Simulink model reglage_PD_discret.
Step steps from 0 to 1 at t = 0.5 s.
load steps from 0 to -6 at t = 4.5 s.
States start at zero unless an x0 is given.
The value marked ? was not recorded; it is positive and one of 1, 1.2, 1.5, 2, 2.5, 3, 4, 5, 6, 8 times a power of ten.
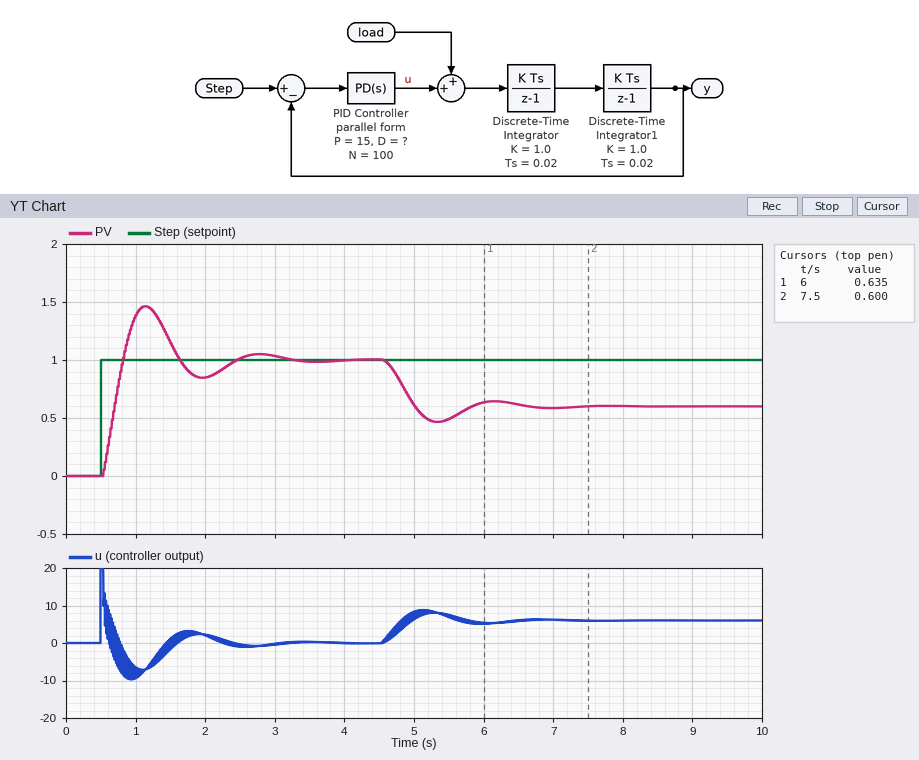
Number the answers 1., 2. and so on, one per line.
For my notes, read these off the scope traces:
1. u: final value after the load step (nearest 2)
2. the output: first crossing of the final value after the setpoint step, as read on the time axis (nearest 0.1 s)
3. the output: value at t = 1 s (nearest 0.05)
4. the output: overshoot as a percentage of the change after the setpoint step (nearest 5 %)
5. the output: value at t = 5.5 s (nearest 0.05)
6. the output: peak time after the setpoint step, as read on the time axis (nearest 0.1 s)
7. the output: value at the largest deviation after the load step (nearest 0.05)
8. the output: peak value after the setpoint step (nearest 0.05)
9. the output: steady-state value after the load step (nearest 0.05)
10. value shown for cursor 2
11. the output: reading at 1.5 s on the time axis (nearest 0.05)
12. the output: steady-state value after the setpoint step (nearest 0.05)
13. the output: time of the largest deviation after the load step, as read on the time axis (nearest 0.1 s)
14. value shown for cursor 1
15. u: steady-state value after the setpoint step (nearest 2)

1. 6
2. 0.8 s
3. 1.40
4. 45 %
5. 0.50
6. 1.1 s
7. 0.45
8. 1.45
9. 0.60
10. 0.600
11. 1.15
12. 1.00
13. 5.3 s
14. 0.635
15. 0
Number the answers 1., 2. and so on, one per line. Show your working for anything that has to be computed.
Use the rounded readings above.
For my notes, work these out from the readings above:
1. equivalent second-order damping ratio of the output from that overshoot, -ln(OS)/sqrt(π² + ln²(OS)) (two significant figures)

1. ln(0.45) = -0.799; 0.799 / sqrt(9.870 + 0.638) = 0.25
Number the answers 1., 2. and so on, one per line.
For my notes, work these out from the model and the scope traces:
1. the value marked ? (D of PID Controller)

1. 1.2
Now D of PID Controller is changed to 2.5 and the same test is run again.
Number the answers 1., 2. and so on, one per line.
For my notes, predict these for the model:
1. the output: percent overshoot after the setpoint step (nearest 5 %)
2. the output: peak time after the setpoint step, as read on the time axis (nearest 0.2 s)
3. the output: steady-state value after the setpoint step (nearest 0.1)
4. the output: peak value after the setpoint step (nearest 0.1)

1. 25 %
2. 1.0 s
3. 1.0
4. 1.2
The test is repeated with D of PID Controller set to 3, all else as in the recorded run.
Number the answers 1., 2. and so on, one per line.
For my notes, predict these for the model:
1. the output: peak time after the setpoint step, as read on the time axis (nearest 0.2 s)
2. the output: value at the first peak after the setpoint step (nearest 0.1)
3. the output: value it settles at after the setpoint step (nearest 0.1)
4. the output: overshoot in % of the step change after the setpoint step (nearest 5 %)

1. 1.0 s
2. 1.2
3. 1.0
4. 20 %
